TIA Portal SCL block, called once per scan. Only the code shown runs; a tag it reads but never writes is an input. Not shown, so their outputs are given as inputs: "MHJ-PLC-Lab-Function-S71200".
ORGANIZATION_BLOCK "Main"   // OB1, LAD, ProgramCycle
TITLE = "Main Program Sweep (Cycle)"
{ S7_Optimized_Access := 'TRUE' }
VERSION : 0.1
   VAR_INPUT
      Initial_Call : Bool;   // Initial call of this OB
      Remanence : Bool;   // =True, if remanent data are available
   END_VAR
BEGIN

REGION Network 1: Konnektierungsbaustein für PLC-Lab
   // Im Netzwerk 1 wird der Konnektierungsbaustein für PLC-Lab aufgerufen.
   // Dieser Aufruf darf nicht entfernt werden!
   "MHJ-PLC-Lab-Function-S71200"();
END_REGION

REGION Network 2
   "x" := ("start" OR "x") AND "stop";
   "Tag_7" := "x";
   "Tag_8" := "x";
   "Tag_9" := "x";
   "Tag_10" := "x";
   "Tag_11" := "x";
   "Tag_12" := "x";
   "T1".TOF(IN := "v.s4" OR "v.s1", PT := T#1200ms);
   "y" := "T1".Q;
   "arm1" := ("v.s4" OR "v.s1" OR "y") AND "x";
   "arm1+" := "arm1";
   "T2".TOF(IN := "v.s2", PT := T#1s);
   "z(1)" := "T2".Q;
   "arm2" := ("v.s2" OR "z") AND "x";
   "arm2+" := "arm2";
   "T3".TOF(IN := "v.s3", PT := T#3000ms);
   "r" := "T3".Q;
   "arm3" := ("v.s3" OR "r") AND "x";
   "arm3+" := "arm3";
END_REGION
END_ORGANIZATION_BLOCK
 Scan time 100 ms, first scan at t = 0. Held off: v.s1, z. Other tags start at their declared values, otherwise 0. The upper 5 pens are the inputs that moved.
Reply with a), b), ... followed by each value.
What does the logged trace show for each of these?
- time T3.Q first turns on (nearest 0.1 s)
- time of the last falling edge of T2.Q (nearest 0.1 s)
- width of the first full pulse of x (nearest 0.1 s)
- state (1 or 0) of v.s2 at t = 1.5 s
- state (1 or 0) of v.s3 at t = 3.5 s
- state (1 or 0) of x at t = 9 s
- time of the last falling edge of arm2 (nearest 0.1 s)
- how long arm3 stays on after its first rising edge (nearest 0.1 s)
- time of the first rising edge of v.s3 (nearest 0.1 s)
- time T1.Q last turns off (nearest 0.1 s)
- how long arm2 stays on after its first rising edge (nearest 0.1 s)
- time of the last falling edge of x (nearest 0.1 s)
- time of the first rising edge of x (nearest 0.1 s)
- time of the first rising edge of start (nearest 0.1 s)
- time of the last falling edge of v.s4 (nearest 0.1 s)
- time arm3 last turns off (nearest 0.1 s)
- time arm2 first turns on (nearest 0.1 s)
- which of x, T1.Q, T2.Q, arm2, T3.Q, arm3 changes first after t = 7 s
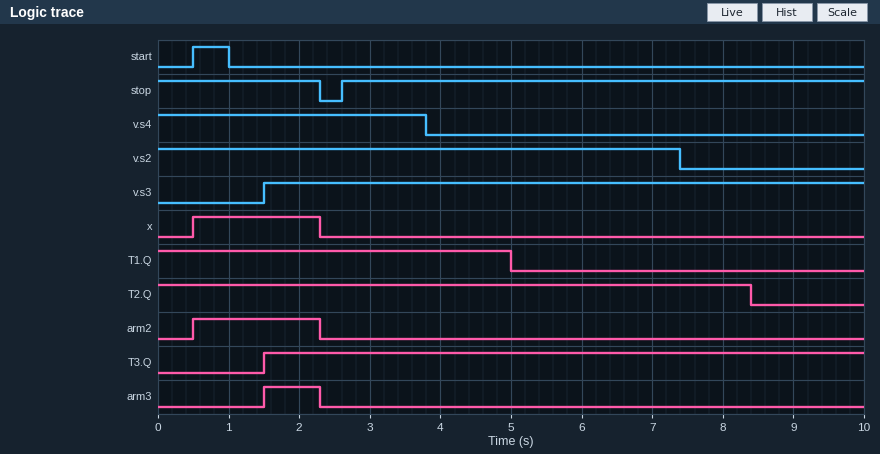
a) 1.5 s
b) 8.4 s
c) 1.8 s
d) 1
e) 1
f) 0
g) 2.3 s
h) 0.8 s
i) 1.5 s
j) 5.0 s
k) 1.8 s
l) 2.3 s
m) 0.5 s
n) 0.5 s
o) 3.8 s
p) 2.3 s
q) 0.5 s
r) T2.Q
